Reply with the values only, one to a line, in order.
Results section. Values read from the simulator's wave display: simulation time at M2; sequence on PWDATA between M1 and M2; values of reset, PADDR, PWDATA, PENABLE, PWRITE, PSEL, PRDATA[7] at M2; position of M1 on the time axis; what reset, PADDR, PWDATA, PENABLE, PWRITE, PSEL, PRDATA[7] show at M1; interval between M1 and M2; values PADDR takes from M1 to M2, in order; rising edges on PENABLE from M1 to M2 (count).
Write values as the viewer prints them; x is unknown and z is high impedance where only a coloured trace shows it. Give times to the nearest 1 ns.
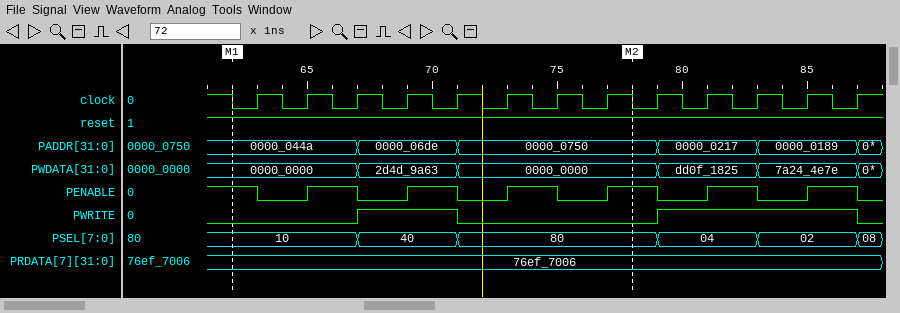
78 ns
0000_0000, 2d4d_9a63, 0000_0000
reset=1, PADDR=0000_0750, PWDATA=0000_0000, PENABLE=1, PWRITE=0, PSEL=80, PRDATA[7]=76ef_7006
62 ns
reset=1, PADDR=0000_044a, PWDATA=0000_0000, PENABLE=1, PWRITE=0, PSEL=10, PRDATA[7]=76ef_7006
16 ns
0000_044a, 0000_06de, 0000_0750
4
